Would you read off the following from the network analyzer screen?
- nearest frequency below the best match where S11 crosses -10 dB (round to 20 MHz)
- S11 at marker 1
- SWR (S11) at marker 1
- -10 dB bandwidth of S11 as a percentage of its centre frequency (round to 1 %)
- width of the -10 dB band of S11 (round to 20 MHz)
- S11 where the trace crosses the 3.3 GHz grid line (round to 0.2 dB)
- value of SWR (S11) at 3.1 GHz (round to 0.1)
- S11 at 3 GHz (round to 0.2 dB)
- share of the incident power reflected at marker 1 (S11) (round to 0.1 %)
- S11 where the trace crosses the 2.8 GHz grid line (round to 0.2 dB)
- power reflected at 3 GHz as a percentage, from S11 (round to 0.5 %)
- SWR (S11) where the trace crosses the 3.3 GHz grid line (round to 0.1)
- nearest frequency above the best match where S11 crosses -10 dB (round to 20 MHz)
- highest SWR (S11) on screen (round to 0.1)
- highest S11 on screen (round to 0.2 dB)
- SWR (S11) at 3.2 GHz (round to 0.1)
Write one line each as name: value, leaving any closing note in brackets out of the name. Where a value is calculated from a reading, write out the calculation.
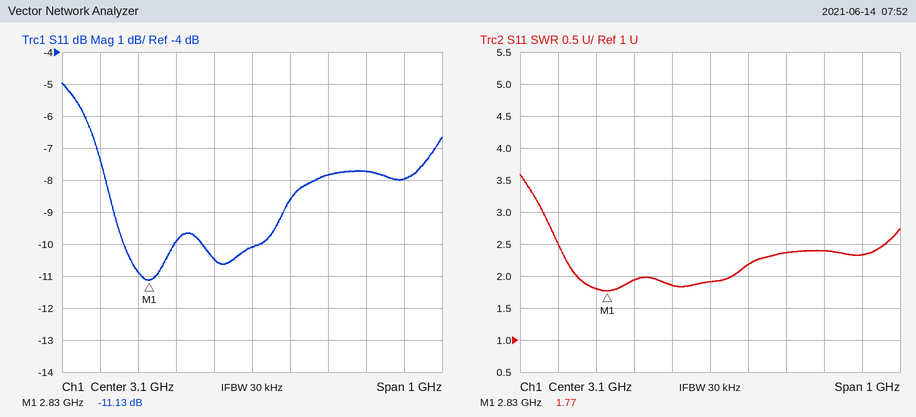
nearest frequency below the best match where S11 crosses -10 dB: 2.76 GHz
S11 at marker 1: -11.13 dB
SWR (S11) at marker 1: 1.77
-10 dB bandwidth of S11 as a percentage of its centre frequency: 140 MHz / 2.83 GHz ≈ 5 %
width of the -10 dB band of S11: 2.90 GHz − 2.76 GHz = 140 MHz
S11 where the trace crosses the 3.3 GHz grid line: -7.8 dB
value of SWR (S11) at 3.1 GHz: 1.9
S11 at 3 GHz: -10.4 dB
share of the incident power reflected at marker 1 (S11): 10^(-11.13/10) ≈ 7.7 %
S11 where the trace crosses the 2.8 GHz grid line: -10.8 dB
power reflected at 3 GHz as a percentage, from S11: 10^(-10.4/10) ≈ 9.12 %, so 9.0 % to the nearest 0.5 %
SWR (S11) where the trace crosses the 3.3 GHz grid line: 2.4
nearest frequency above the best match where S11 crosses -10 dB: 2.90 GHz
highest SWR (S11) on screen: 3.6
highest S11 on screen: -5.0 dB
SWR (S11) at 3.2 GHz: 2.2
